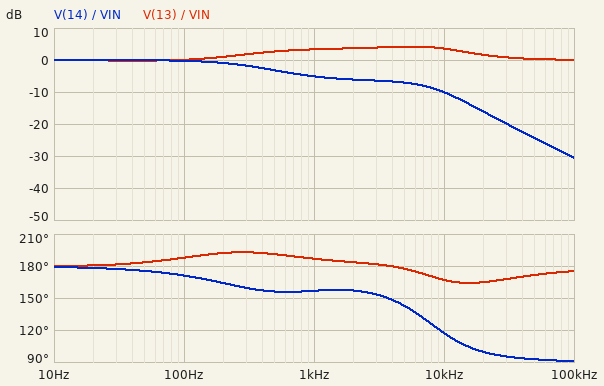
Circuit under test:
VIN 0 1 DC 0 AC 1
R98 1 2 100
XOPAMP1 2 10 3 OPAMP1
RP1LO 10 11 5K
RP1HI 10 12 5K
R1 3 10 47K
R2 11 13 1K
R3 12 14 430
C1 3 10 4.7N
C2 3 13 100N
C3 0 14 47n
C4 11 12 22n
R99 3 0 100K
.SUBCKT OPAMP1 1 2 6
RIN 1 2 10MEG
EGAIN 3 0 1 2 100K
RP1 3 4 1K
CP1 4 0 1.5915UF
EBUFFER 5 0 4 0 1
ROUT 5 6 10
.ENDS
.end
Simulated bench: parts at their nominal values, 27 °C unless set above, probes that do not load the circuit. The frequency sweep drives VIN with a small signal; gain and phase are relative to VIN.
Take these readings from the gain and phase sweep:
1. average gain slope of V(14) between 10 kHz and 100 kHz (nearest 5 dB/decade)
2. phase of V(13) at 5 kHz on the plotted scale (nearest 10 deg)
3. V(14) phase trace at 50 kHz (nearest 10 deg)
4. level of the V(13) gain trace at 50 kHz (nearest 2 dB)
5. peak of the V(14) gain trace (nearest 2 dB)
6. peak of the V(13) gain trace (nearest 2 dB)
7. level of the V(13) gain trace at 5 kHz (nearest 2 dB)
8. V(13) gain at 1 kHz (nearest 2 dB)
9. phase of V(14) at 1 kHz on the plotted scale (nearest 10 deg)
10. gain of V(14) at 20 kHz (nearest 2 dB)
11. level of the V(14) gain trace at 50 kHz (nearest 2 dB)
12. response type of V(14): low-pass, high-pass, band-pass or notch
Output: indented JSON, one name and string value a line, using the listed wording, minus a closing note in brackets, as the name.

{
  "average gain slope of V(14) between 10 kHz and 100 kHz": "-20 dB/decade",
  "phase of V(13) at 5 kHz on the plotted scale": "180 deg",
  "V(14) phase trace at 50 kHz": "90 deg",
  "level of the V(13) gain trace at 50 kHz": "0 dB",
  "peak of the V(14) gain trace": "0 dB",
  "peak of the V(13) gain trace": "4 dB",
  "level of the V(13) gain trace at 5 kHz": "4 dB",
  "V(13) gain at 1 kHz": "4 dB",
  "phase of V(14) at 1 kHz on the plotted scale": "160 deg",
  "gain of V(14) at 20 kHz": "-16 dB",
  "level of the V(14) gain trace at 50 kHz": "-24 dB",
  "response type of V(14): low-pass, high-pass, band-pass or notch": "low-pass"
}
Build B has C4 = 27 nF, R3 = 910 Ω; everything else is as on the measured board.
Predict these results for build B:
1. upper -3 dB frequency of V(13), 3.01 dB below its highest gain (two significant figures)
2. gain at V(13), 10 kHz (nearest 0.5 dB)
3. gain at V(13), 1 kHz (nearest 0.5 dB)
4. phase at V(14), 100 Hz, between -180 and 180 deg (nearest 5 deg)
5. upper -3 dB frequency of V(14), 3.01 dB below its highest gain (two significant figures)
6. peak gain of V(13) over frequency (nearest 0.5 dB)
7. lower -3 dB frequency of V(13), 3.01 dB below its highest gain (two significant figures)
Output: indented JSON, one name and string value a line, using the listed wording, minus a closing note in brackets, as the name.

{
  "upper -3 dB frequency of V(13), 3.01 dB below its highest gain": "30 kHz",
  "gain at V(13), 10 kHz": "2.5 dB",
  "gain at V(13), 1 kHz": "3.0 dB",
  "phase at V(14), 100 Hz, between -180 and 180 deg": "170 deg",
  "upper -3 dB frequency of V(14), 3.01 dB below its highest gain": "440 Hz",
  "peak gain of V(13) over frequency": "3.5 dB",
  "lower -3 dB frequency of V(13), 3.01 dB below its highest gain": "140 Hz"
}
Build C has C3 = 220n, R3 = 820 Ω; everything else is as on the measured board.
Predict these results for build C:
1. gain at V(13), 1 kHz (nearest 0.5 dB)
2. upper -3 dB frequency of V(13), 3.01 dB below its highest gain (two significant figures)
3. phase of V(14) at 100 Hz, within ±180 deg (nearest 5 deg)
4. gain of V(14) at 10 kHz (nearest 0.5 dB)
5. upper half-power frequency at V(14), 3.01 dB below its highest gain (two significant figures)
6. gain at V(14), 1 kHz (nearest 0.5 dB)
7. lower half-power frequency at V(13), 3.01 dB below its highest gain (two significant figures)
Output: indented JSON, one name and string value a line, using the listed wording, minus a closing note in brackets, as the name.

{
  "gain at V(13), 1 kHz": "5.0 dB",
  "upper -3 dB frequency of V(13), 3.01 dB below its highest gain": "13 kHz",
  "phase of V(14) at 100 Hz, within ±180 deg": "145 deg",
  "gain of V(14) at 10 kHz": "-25.5 dB",
  "upper half-power frequency at V(14), 3.01 dB below its highest gain": "110 Hz",
  "gain at V(14), 1 kHz": "-15.0 dB",
  "lower half-power frequency at V(13), 3.01 dB below its highest gain": "86 Hz"
}
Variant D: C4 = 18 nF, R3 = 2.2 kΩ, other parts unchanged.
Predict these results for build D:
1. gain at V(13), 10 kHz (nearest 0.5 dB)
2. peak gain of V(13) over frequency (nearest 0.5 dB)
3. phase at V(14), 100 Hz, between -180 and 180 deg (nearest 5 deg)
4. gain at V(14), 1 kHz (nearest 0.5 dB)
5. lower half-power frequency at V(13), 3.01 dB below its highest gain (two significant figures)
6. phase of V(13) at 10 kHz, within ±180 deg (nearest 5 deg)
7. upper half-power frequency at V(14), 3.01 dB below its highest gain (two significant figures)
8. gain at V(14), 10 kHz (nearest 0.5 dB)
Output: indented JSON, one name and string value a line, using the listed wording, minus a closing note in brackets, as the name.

{
  "gain at V(13), 10 kHz": "1.0 dB",
  "peak gain of V(13) over frequency": "3.5 dB",
  "phase at V(14), 100 Hz, between -180 and 180 deg": "170 deg",
  "gain at V(14), 1 kHz": "-6.5 dB",
  "lower half-power frequency at V(13), 3.01 dB below its highest gain": "120 Hz",
  "phase of V(13) at 10 kHz, within ±180 deg": "170 deg",
  "upper half-power frequency at V(14), 3.01 dB below its highest gain": "390 Hz",
  "gain at V(14), 10 kHz": "-18.5 dB"
}
